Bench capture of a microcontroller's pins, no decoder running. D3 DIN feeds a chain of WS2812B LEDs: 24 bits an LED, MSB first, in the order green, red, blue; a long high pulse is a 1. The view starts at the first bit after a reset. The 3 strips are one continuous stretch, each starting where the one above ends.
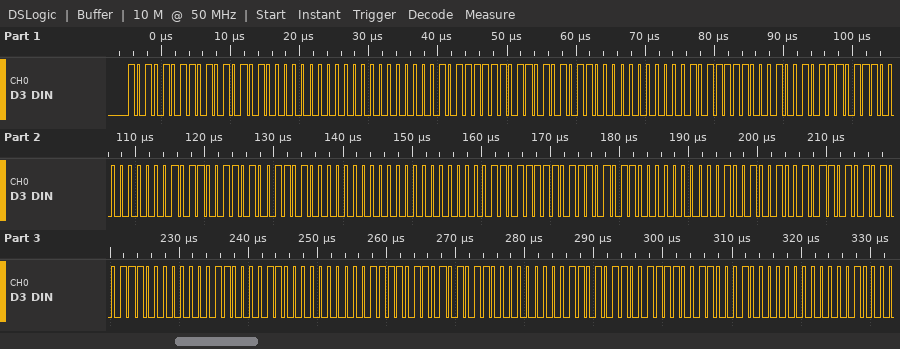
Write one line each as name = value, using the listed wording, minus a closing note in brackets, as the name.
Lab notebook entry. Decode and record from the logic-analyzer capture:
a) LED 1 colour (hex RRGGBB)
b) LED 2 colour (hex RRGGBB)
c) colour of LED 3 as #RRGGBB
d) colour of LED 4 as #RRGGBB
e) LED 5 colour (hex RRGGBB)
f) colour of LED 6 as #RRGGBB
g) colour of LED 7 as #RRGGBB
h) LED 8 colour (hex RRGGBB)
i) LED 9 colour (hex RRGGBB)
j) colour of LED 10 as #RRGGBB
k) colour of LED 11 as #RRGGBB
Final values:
LED 1 colour = #55AB00
LED 2 colour = #0B00F6
colour of LED 3 as #RRGGBB = #00AC5F
colour of LED 4 as #RRGGBB = #EE1200
LED 5 colour = #4DB300
colour of LED 6 as #RRGGBB = #0600FB
colour of LED 7 as #RRGGBB = #00AC92
LED 8 colour = #A75A00
LED 9 colour = #00C33D
colour of LED 10 as #RRGGBB = #00AB6B
colour of LED 11 as #RRGGBB = #C43C00
